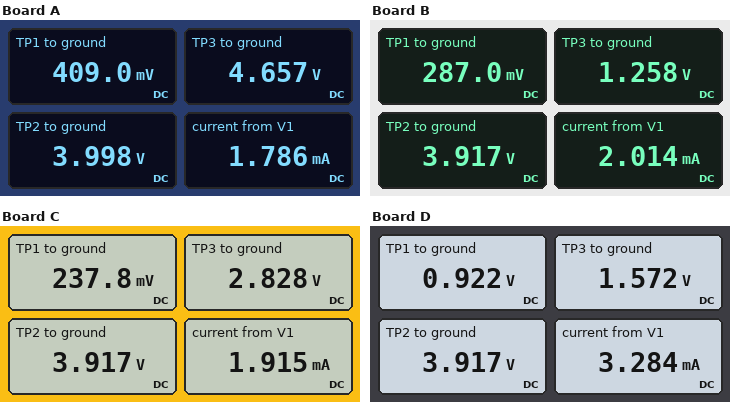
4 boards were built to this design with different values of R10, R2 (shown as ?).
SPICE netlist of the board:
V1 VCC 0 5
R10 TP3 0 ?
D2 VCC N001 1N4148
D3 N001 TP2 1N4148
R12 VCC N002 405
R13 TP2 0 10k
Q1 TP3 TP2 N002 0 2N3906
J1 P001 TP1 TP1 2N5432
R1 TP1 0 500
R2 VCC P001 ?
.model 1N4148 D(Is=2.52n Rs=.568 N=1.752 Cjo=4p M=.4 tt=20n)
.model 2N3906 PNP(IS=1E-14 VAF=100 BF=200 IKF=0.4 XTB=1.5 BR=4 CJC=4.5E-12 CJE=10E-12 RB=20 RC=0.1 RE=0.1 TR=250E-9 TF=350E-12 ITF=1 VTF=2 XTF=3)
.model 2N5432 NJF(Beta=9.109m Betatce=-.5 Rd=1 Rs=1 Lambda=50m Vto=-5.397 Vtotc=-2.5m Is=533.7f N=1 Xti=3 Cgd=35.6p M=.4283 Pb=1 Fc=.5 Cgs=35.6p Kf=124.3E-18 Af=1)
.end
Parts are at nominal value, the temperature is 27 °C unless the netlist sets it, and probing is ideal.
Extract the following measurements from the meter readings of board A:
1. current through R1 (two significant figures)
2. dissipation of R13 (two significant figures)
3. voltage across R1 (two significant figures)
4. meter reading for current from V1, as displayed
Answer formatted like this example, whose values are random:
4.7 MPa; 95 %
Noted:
820 µA; 1.6 mW; 410 mV; 1.786 mA
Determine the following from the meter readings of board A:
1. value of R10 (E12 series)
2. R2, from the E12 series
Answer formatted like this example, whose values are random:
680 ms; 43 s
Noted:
8.2 kΩ; 5.6 kΩ
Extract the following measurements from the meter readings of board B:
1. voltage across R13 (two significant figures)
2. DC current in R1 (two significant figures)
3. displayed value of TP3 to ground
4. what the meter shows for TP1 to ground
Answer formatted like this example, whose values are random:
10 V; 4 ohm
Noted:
3.9 V; 570 µA; 1.258 V; 287.0 mV
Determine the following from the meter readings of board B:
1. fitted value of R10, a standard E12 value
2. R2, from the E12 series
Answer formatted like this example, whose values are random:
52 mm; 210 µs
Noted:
1.2 kΩ; 8.2 kΩ
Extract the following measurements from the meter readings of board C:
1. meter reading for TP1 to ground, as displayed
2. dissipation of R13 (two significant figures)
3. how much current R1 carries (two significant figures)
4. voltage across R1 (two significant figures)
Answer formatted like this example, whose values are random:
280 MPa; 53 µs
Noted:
237.8 mV; 1.5 mW; 480 µA; 240 mV
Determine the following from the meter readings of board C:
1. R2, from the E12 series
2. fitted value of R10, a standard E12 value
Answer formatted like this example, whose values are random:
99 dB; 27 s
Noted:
10 kΩ; 2.7 kΩ
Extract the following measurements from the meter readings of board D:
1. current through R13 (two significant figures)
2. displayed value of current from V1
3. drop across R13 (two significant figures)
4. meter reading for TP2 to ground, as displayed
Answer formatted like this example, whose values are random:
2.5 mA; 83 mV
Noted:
390 µA; 3.284 mA; 3.9 V; 3.917 V
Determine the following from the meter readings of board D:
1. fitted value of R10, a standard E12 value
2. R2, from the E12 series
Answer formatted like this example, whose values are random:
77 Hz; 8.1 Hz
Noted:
1.5 kΩ; 2.2 kΩ
